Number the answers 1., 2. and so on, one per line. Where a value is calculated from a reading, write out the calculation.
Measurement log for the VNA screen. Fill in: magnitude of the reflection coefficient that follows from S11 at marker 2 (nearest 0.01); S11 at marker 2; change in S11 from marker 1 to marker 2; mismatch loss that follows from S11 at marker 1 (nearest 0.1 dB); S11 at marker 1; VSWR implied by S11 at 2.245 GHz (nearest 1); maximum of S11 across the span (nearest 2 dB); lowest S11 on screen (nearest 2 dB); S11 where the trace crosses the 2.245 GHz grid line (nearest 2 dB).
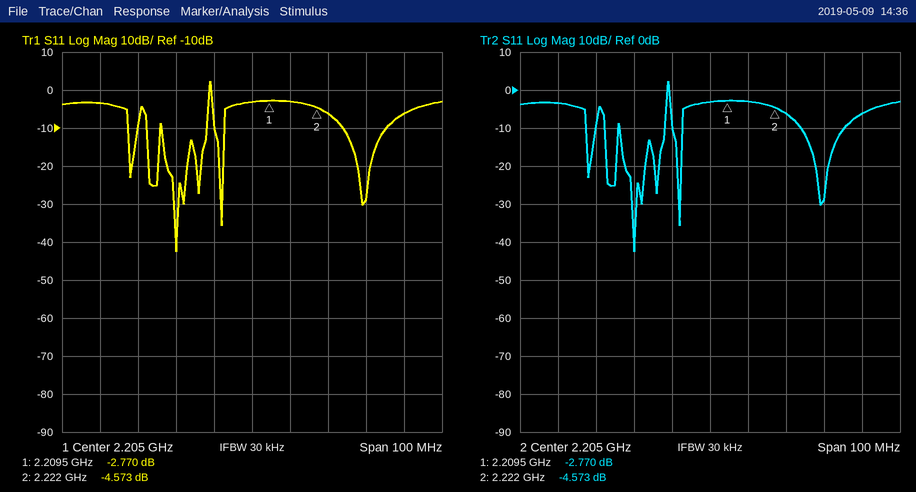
1. 10^(-4.573/20) ≈ 0.59
2. -4.573 dB
3. -4.573 − (-2.77) = -1.803 dB
4. −10 log10(1 − 10^(-2.77/10)) ≈ 3.3 dB
5. -2.770 dB
6. |Γ| = 10^(-6/20) = 0.5012; VSWR = (1 + 0.5012)/(1 − 0.5012) ≈ 3
7. 2 dB
8. -42 dB
9. -6 dB
